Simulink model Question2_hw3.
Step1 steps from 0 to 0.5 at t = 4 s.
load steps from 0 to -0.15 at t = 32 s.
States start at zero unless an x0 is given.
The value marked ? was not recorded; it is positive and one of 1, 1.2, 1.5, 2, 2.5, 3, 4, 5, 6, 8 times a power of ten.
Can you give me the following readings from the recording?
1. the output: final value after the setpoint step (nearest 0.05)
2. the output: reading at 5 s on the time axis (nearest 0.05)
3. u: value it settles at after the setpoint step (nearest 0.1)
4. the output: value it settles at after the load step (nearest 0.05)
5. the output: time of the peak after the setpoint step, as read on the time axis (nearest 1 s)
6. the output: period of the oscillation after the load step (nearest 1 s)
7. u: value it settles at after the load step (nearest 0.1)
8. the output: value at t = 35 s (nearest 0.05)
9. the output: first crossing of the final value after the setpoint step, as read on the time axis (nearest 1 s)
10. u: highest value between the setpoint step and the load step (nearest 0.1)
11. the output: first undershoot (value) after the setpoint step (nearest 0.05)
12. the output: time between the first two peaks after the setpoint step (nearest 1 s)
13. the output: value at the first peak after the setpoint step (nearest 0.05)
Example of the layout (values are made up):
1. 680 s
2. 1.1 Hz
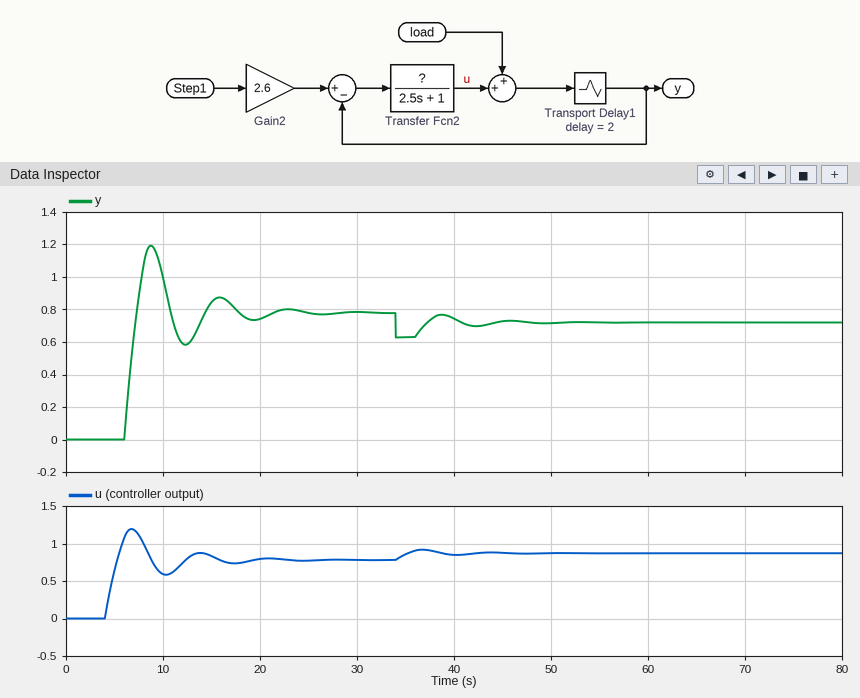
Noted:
1. 0.80
2. 0.00
3. 0.8
4. 0.70
5. 9 s
6. 8 s
7. 0.9
8. 0.65
9. 7 s
10. 1.2
11. 0.60
12. 7 s
13. 1.20
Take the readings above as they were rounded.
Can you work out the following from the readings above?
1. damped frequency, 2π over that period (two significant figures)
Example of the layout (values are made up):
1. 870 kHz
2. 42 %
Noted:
1. 0.90 rad/s
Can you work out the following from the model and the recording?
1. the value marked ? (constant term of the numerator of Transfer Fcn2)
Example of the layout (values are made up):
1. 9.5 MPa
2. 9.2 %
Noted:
1. 1.5
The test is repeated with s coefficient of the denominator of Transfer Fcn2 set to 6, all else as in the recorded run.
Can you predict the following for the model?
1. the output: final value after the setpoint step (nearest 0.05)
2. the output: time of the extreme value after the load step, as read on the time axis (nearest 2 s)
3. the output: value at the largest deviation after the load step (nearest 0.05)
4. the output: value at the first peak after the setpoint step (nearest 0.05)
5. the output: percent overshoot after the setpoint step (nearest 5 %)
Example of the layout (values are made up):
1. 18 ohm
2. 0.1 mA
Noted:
1. 0.80
2. 36 s
3. 0.65
4. 0.85
5. 10 %
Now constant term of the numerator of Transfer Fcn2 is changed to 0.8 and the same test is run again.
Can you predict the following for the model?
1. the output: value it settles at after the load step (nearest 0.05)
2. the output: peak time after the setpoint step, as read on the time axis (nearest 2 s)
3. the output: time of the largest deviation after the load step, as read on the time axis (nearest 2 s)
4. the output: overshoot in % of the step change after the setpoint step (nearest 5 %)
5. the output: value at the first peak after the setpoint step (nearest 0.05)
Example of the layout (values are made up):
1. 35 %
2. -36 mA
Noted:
1. 0.50
2. 10 s
3. 36 s
4. 20 %
5. 0.70
